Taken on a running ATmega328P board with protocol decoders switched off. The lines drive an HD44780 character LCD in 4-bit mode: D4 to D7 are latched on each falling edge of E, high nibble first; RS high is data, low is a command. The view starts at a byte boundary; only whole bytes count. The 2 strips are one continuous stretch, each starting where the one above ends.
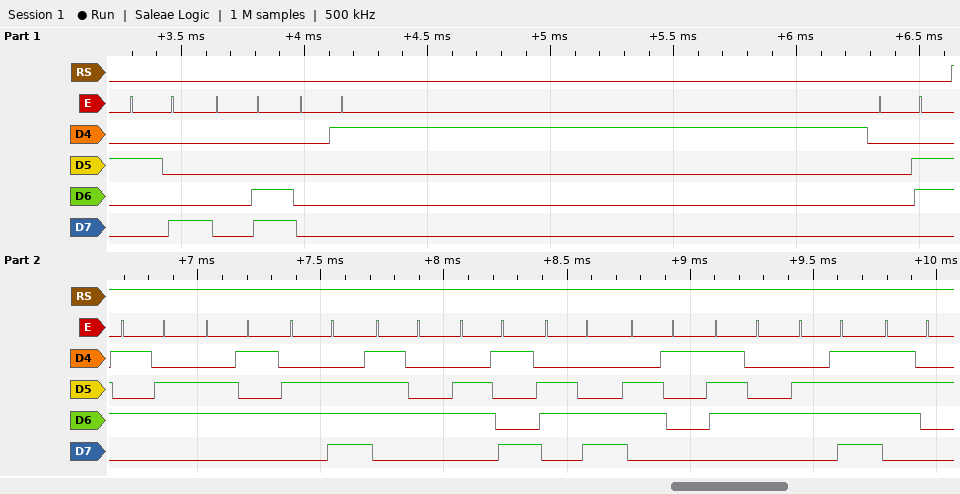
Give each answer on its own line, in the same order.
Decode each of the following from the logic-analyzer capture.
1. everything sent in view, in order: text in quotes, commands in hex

0x28 0x0C 0x01 0x06 "Ventilator"
